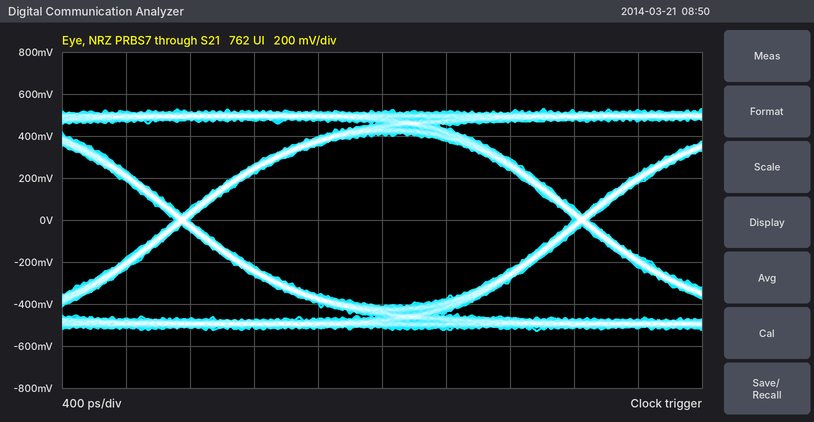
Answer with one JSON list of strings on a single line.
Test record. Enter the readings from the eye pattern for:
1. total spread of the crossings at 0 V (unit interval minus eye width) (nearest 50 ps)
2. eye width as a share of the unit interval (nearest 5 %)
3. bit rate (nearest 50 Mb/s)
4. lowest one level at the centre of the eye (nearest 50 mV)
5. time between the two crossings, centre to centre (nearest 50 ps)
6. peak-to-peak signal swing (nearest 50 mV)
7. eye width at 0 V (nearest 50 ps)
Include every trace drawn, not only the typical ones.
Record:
["100 ps", "95 %", "400 Mb/s", "400 mV", "2.50 ns", "1.05 V", "2.40 ns"]
